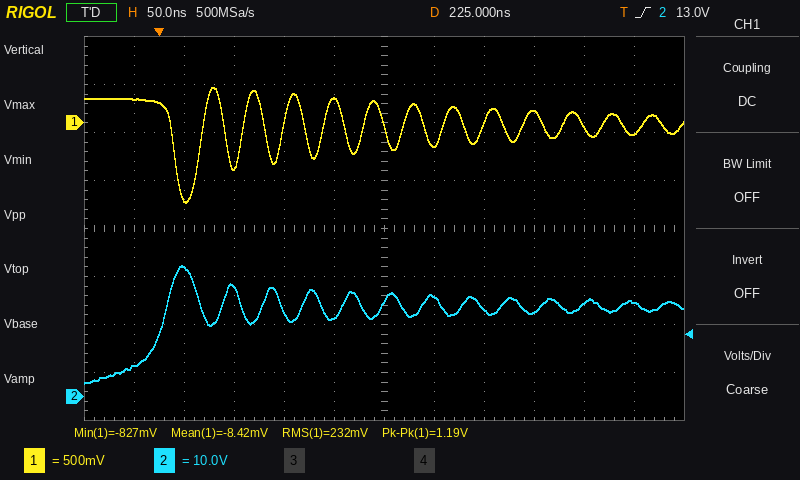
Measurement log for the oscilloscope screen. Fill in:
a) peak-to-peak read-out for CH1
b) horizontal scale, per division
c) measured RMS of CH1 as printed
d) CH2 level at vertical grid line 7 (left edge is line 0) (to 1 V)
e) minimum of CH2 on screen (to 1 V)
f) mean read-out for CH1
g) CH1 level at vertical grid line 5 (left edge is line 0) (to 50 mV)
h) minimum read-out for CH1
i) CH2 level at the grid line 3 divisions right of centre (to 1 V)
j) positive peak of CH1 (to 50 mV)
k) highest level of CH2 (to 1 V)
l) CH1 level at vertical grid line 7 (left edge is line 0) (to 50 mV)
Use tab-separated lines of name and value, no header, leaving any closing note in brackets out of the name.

peak-to-peak read-out for CH1	1.19 V
horizontal scale, per division	50 ns
measured RMS of CH1 as printed	232 mV
CH2 level at vertical grid line 7 (left edge is line 0)	21 V
minimum of CH2 on screen	3 V
mean read-out for CH1	-8.42 mV
CH1 level at vertical grid line 5 (left edge is line 0)	250 mV
minimum read-out for CH1	-827 mV
CH2 level at the grid line 3 divisions right of centre	18 V
positive peak of CH1	350 mV
highest level of CH2	27 V
CH1 level at vertical grid line 7 (left edge is line 0)	-250 mV
